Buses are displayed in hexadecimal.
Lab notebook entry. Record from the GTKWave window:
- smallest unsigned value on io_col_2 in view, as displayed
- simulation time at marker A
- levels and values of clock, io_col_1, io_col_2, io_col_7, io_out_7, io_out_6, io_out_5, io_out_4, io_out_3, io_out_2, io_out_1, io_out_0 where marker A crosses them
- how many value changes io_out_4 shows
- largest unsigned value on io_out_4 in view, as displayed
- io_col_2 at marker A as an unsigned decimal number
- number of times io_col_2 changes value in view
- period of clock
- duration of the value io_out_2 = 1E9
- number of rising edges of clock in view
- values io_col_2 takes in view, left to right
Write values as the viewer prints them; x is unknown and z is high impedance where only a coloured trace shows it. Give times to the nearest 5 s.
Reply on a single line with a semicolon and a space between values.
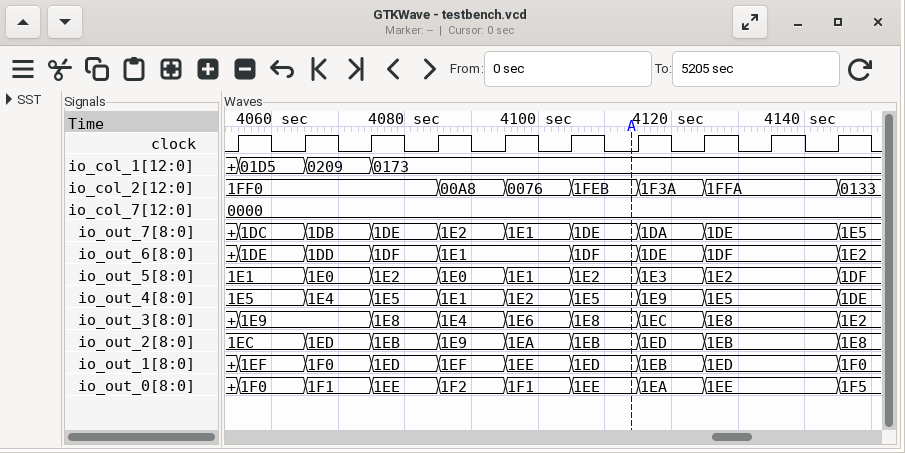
0076; 4115 s; clock=0, io_col_1=0173, io_col_2=1FEB, io_col_7=0000, io_out_7=1DE, io_out_6=1DF, io_out_5=1E2, io_out_4=1E5, io_out_3=1E8, io_out_2=1EB, io_out_1=1ED, io_out_0=1EE; 8; 1E9; 8171; 6; 10 s; 10 s; 10; 1FF0, 00A8, 0076, 1FEB, 1F3A, 1FFA, 0133
